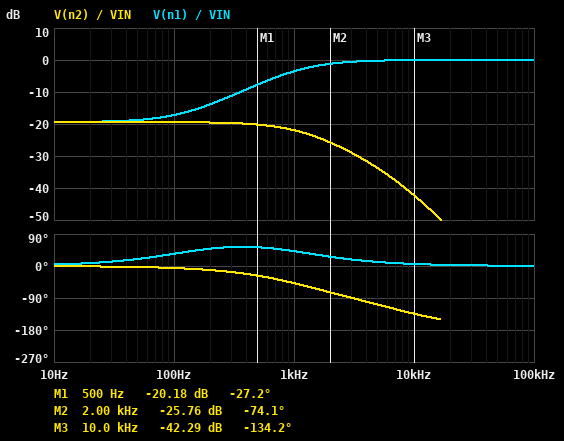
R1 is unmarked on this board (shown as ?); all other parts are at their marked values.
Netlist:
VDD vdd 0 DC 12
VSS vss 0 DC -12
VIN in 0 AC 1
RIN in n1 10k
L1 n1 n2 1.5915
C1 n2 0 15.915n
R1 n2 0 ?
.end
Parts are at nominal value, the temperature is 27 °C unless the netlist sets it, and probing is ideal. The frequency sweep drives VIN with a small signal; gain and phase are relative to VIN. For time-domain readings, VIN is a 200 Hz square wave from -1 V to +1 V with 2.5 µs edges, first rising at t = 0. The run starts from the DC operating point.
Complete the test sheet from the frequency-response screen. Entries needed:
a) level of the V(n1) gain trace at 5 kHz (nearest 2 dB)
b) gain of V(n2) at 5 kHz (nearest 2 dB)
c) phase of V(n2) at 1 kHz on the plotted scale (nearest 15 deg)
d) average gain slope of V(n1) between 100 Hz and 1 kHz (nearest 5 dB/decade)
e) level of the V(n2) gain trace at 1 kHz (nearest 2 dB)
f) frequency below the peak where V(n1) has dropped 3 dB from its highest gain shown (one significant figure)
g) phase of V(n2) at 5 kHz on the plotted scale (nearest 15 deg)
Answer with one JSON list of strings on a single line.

["0 dB", "-34 dB", "-45 deg", "15 dB/decade", "-22 dB", "1 kHz", "-105 deg"]
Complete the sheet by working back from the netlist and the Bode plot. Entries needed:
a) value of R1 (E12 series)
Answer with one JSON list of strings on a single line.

["1.2 kΩ"]
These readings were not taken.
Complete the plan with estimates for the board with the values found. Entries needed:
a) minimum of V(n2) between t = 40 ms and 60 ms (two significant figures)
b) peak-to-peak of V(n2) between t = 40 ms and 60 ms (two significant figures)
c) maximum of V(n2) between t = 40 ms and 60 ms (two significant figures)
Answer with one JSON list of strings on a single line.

["-110 mV", "210 mV", "110 mV"]
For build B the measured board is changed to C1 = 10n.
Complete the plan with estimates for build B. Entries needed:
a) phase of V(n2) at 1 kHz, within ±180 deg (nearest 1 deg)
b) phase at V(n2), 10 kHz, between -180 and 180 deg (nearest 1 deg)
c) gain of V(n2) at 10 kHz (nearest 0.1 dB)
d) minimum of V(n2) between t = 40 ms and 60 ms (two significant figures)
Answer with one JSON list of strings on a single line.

["-46 deg", "-121 deg", "-40.4 dB", "-110 mV"]
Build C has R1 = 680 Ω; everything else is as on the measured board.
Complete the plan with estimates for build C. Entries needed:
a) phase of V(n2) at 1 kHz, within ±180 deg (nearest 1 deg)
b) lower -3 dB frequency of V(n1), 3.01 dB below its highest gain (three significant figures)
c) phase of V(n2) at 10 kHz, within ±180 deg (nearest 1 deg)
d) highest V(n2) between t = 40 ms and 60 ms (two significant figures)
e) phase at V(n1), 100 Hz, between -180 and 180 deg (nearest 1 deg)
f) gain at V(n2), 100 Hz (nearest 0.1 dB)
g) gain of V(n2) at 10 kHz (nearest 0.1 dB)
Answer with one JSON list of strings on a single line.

["-47 deg", "1.07 kHz", "-118 deg", "64 mV", "50 deg", "-24.0 dB", "-45.0 dB"]
